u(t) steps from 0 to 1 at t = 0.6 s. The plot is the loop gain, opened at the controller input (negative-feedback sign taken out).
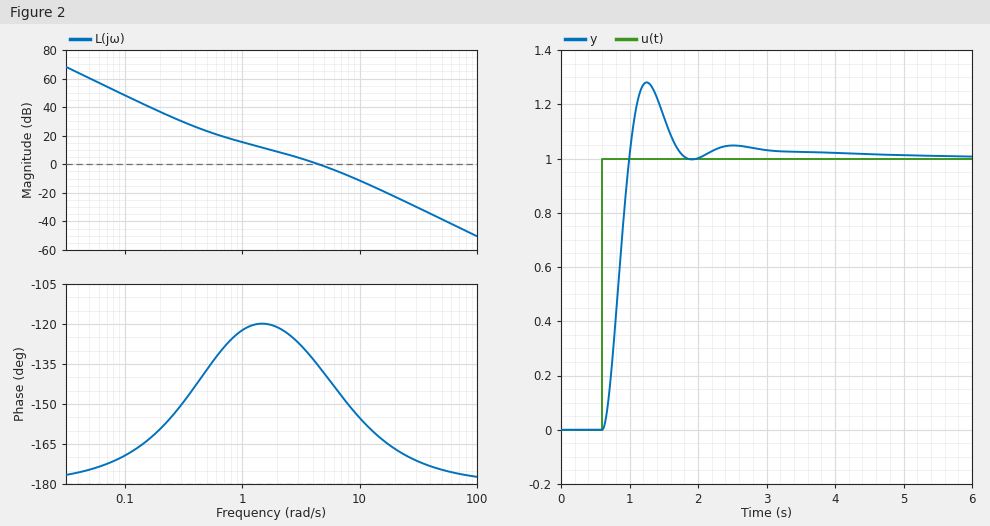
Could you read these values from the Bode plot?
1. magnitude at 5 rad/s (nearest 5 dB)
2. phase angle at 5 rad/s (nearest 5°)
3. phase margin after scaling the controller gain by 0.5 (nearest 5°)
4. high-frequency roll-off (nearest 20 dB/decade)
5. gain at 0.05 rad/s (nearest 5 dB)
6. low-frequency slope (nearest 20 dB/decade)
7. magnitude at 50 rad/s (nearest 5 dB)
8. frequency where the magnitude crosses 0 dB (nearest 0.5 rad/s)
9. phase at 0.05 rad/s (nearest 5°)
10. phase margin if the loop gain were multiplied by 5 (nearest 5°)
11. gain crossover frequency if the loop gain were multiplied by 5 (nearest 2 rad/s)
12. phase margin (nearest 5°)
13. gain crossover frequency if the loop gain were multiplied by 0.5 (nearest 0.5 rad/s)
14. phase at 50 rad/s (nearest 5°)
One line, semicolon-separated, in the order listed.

0 dB; -140°; 55°; -40 dB/decade; 60 dB; -40 dB/decade; -40 dB; 4.5 rad/s; -175°; 20°; 12 rad/s; 45°; 2.5 rad/s; -175°
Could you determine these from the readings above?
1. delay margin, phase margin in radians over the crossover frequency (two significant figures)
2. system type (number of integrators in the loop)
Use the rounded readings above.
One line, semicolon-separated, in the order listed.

0.17 s; 2
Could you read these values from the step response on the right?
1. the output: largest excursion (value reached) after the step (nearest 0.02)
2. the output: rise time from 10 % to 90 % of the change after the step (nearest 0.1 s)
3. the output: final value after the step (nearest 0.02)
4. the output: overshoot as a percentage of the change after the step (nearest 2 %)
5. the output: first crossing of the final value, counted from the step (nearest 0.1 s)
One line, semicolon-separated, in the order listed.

1.28; 0.3 s; 1.00; 28 %; 0.4 s
